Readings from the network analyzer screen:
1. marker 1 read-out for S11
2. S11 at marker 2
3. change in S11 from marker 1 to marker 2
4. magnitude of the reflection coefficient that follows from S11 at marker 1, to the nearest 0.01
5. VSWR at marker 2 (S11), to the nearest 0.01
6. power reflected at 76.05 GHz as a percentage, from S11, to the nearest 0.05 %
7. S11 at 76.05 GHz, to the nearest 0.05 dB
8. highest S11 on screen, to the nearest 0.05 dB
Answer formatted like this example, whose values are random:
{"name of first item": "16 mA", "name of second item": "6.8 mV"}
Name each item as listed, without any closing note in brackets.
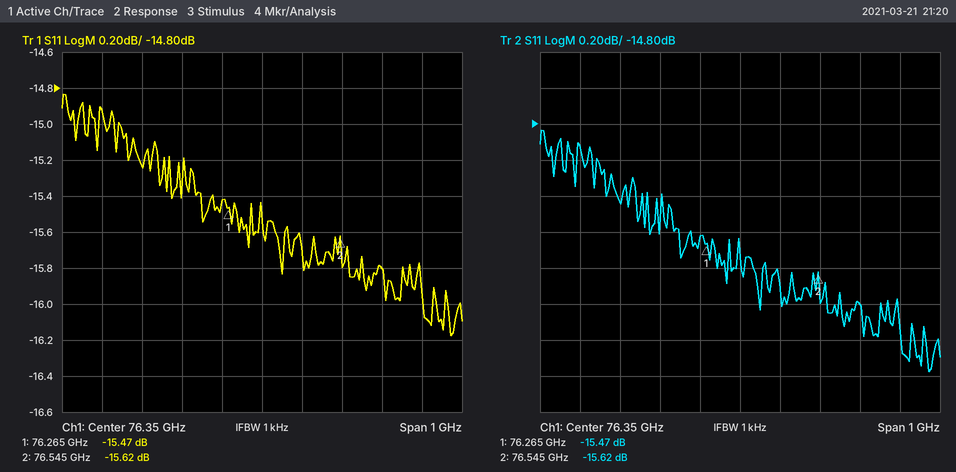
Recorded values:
{"marker 1 read-out for S11": "-15.47 dB", "S11 at marker 2": "-15.62 dB", "change in S11 from marker 1 to marker 2": "-0.15 dB", "magnitude of the reflection coefficient that follows from S11 at marker 1, to the nearest 0.01": "0.17", "VSWR at marker 2 (S11), to the nearest 0.01": "1.40", "power reflected at 76.05 GHz as a percentage, from S11, to the nearest 0.05 %": "3.00 %", "S11 at 76.05 GHz, to the nearest 0.05 dB": "-15.25 dB", "highest S11 on screen, to the nearest 0.05 dB": "-14.85 dB"}
